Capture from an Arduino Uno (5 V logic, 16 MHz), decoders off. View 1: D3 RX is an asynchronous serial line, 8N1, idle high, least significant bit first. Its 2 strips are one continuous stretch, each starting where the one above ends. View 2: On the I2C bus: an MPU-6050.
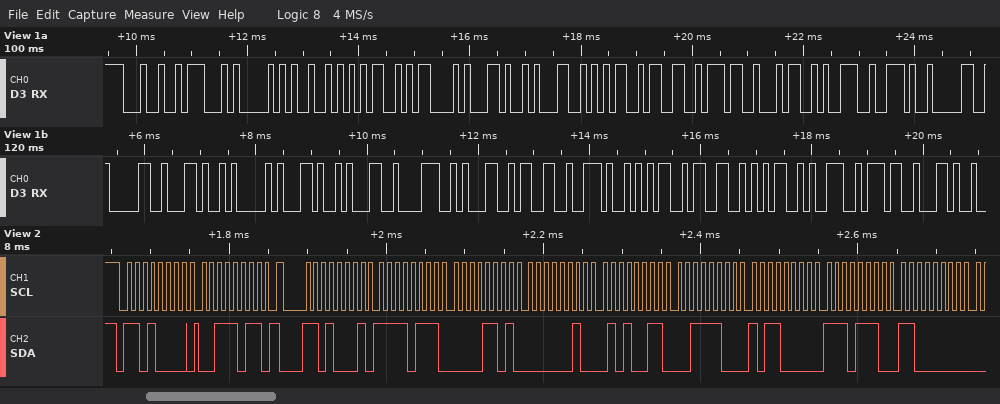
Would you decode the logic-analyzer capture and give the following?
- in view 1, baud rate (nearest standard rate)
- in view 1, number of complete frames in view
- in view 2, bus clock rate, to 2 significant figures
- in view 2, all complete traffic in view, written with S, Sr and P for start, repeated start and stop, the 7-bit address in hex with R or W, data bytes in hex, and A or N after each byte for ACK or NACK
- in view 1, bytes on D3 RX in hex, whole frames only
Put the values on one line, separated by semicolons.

9600 baud; 30; 100 kHz; S 68W A 3B A Sr 68R A F7 A 0D A 02 A 53 A 3C A B0 A EE A C0 A; 24 47 50 52 4D 43 2C 31 35 33 37 34 39 2E 30 30 2C 41 2C 31 38 31 33 2E 35 33 35 39 37 2C
